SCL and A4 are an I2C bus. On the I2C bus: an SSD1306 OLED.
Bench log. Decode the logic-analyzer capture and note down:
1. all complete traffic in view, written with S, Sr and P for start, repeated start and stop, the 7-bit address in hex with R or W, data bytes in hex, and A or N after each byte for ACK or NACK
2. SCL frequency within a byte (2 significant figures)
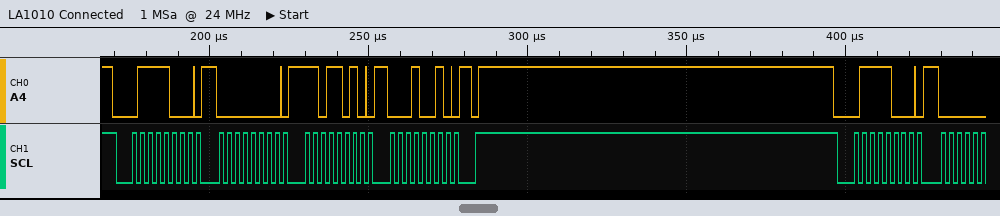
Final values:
S 3CW A 00 A DA A 12 A P S 3CW A
400 kHz
